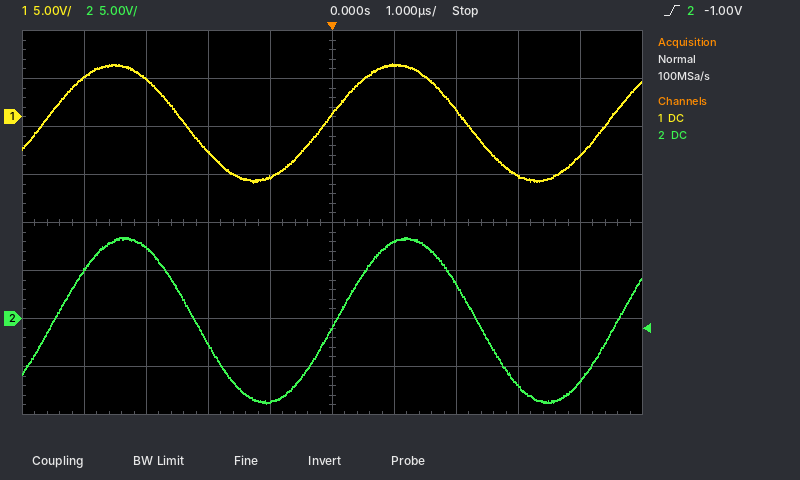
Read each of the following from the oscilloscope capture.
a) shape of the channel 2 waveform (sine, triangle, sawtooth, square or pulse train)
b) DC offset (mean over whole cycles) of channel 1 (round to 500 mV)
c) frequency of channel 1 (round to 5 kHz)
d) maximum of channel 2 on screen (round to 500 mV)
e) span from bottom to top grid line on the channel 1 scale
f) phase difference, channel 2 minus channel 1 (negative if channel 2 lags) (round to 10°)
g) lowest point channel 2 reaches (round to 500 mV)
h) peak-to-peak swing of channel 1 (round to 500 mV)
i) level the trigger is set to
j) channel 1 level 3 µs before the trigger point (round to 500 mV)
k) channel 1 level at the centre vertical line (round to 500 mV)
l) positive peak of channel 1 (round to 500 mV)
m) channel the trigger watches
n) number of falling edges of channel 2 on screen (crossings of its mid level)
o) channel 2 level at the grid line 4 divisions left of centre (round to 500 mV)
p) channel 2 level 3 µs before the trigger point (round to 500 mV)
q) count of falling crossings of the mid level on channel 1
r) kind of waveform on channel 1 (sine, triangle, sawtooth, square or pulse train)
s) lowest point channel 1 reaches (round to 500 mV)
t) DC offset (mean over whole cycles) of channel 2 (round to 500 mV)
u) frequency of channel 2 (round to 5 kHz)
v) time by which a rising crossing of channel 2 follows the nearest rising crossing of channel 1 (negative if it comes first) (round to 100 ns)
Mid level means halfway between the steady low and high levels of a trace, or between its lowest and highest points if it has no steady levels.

sine
-500 mV
220 kHz
8.5 V
40 V
-10°
-9.0 V
12.5 V
-1.00 V
4.0 V
500 mV
5.5 V
channel 2
2
5.0 V
7.5 V
2
sine
-7.0 V
0.0 V
220 kHz
+200 ns
